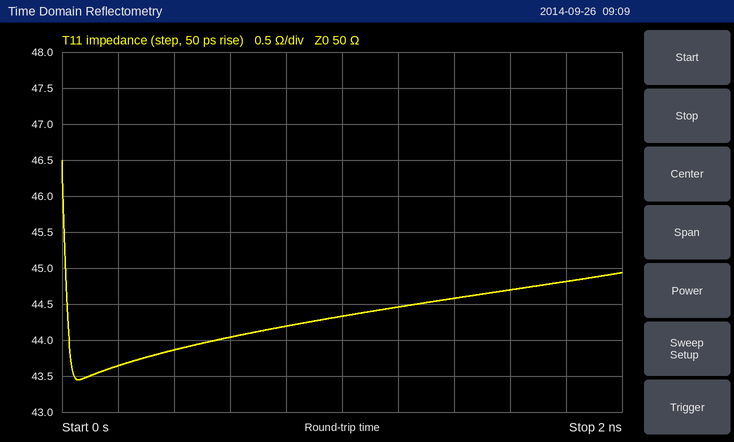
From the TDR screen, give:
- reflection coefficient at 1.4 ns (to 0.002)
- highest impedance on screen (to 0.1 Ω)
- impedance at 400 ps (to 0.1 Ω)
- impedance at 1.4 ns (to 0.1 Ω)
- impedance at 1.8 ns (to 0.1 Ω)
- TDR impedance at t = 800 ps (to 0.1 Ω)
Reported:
-0.058
46.5 Ω
43.9 Ω
44.6 Ω
44.8 Ω
44.2 Ω
